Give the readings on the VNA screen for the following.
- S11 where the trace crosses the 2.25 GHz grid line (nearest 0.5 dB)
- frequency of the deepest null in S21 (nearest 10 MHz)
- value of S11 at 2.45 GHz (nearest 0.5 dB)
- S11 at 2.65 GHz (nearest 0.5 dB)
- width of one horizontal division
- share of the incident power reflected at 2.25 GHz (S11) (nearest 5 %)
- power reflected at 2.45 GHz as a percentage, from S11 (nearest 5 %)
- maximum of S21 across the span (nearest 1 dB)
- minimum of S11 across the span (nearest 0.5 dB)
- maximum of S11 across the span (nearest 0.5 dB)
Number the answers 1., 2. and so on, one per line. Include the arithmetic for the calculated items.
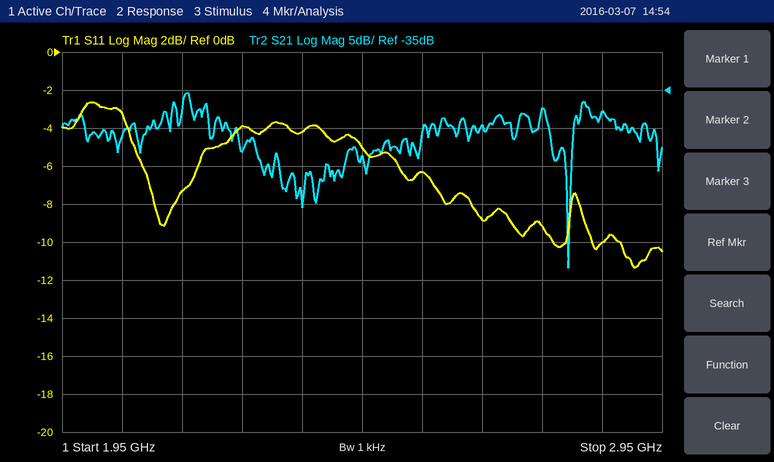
1. -4.0 dB
2. 2.79 GHz
3. -5.0 dB
4. -9.0 dB
5. 100 MHz
6. 10^(-4/10) ≈ 40 %
7. 10^(-5/10) ≈ 31.6 %, so 30 % to the nearest 5 %
8. -35 dB
9. -11.5 dB
10. -2.5 dB
